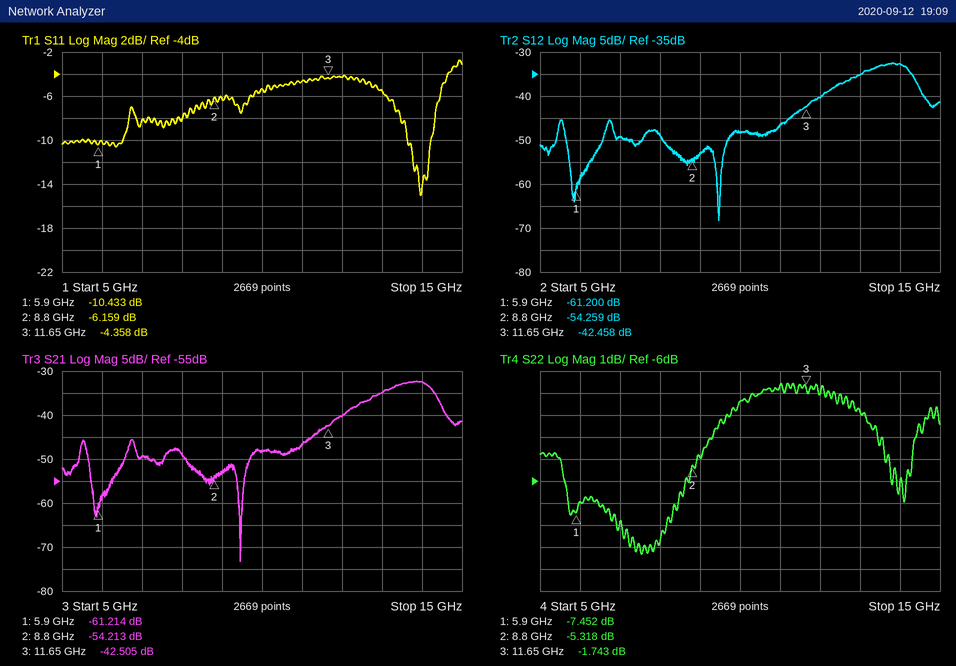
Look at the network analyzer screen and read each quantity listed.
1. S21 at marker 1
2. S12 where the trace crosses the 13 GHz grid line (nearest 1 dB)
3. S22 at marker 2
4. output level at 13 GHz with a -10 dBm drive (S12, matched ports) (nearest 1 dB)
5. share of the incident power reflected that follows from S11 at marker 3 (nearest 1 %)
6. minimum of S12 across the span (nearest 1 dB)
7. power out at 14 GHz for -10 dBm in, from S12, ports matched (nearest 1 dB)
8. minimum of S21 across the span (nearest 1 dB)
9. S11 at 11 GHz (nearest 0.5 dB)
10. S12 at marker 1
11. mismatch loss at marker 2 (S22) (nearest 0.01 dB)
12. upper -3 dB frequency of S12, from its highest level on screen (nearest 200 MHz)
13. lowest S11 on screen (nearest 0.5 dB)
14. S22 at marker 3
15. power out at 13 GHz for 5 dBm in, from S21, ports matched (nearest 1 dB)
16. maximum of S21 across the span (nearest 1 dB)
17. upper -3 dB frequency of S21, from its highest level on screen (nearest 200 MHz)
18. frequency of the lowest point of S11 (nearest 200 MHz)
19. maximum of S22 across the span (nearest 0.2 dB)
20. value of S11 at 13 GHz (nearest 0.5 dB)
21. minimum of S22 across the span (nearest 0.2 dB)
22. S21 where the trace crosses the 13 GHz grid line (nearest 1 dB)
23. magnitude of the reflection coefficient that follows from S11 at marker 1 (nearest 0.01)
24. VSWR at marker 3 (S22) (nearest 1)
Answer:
-61.214 dB
-35 dB
-5.318 dB
-45 dBm
37 %
-68 dB
-43 dBm
-73 dB
-4.5 dB
-61.200 dB
1.51 dB
14.4 GHz
-15.0 dB
-1.743 dB
-30 dBm
-32 dB
14.4 GHz
14.0 GHz
-1.6 dB
-5.5 dB
-9.4 dB
-35 dB
0.30
10
